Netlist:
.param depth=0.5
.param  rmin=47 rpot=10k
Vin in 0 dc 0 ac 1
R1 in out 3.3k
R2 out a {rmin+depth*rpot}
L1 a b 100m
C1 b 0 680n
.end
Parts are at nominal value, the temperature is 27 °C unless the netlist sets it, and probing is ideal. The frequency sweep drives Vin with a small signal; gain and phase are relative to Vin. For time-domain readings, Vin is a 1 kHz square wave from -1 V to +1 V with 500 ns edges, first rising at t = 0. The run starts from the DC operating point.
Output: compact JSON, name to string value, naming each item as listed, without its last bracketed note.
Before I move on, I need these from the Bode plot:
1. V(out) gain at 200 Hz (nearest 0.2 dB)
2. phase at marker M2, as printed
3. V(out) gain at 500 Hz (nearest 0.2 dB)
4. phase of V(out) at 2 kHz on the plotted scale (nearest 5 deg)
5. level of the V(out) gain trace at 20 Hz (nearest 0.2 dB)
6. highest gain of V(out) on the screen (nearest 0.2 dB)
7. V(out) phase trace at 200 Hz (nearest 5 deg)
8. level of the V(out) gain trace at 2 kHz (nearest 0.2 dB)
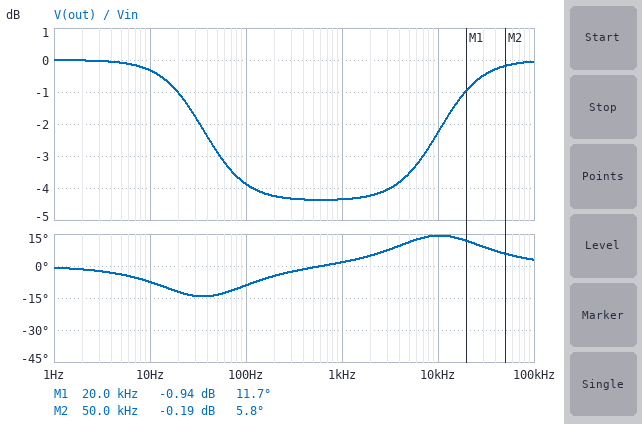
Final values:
{"V(out) gain at 200 Hz": "-4.2 dB", "phase at marker M2, as printed": "5.8 deg", "V(out) gain at 500 Hz": "-4.4 dB", "phase of V(out) at 2 kHz on the plotted scale": "5 deg", "level of the V(out) gain trace at 20 Hz": "-1.0 dB", "highest gain of V(out) on the screen": "0 dB", "V(out) phase trace at 200 Hz": "-5 deg", "level of the V(out) gain trace at 2 kHz": "-4.2 dB"}
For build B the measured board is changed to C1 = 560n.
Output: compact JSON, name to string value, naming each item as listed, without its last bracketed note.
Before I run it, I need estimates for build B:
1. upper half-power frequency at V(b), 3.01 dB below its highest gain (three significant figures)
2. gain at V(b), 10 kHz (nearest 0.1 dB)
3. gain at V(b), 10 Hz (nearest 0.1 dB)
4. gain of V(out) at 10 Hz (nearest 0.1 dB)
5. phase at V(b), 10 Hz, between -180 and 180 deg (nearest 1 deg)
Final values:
{"upper half-power frequency at V(b), 3.01 dB below its highest gain": "34.1 Hz", "gain at V(b), 10 kHz": "-51.3 dB", "gain at V(b), 10 Hz": "-0.4 dB", "gain of V(out) at 10 Hz": "-0.2 dB", "phase at V(b), 10 Hz, between -180 and 180 deg": "-16 deg"}
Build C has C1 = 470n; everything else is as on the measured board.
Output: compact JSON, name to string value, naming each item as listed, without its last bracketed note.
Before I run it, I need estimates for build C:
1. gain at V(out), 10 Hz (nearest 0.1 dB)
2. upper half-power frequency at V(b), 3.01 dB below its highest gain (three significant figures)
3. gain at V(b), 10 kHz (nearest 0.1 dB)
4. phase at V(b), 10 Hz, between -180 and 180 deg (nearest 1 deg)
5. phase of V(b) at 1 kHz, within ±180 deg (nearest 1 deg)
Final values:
{"gain at V(out), 10 Hz": "-0.2 dB", "upper half-power frequency at V(b), 3.01 dB below its highest gain": "40.7 Hz", "gain at V(b), 10 kHz": "-49.8 dB", "phase at V(b), 10 Hz, between -180 and 180 deg": "-14 deg", "phase of V(b) at 1 kHz, within ±180 deg": "-92 deg"}
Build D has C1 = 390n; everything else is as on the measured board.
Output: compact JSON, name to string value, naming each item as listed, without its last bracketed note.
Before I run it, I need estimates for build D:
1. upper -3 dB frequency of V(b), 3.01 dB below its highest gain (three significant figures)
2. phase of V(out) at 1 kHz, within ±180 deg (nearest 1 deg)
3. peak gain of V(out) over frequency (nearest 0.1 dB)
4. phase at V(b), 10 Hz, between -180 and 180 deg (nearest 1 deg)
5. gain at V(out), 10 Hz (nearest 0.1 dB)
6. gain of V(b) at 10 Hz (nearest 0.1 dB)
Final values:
{"upper -3 dB frequency of V(b), 3.01 dB below its highest gain": "49.1 Hz", "phase of V(out) at 1 kHz, within ±180 deg": "1 deg", "peak gain of V(out) over frequency": "0 dB", "phase at V(b), 10 Hz, between -180 and 180 deg": "-12 deg", "gain at V(out), 10 Hz": "-0.1 dB", "gain of V(b) at 10 Hz": "-0.2 dB"}
